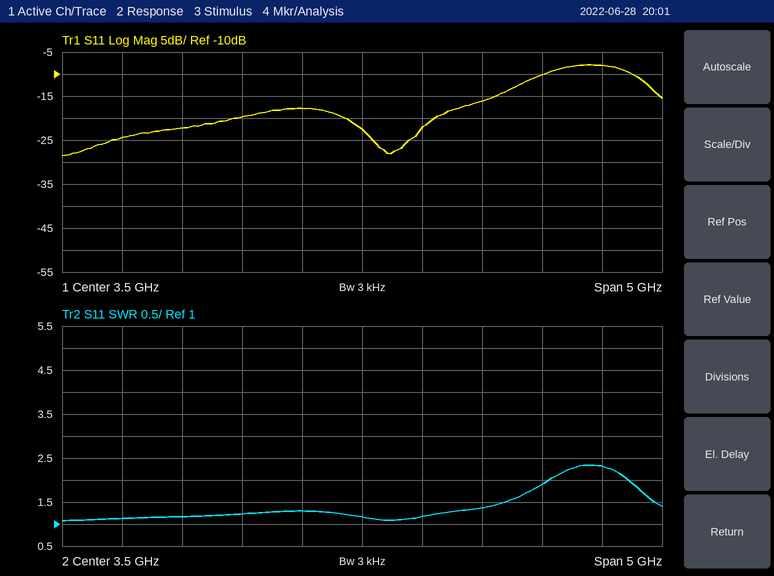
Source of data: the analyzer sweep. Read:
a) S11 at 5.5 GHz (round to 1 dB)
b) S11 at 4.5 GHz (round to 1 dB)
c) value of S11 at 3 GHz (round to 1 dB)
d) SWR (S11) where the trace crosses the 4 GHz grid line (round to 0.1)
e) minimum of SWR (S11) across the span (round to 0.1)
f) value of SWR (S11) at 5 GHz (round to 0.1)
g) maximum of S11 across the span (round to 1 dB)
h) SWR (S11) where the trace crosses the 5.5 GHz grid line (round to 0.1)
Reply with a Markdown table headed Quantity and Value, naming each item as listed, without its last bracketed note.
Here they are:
| Quantity | Value |
|---|---|
| S11 at 5.5 GHz | -8 dB |
| S11 at 4.5 GHz | -16 dB |
| value of S11 at 3 GHz | -18 dB |
| SWR (S11) where the trace crosses the 4 GHz grid line | 1.2 |
| minimum of SWR (S11) across the span | 1.1 |
| value of SWR (S11) at 5 GHz | 1.9 |
| maximum of S11 across the span | -8 dB |
| SWR (S11) where the trace crosses the 5.5 GHz grid line | 2.3 |
